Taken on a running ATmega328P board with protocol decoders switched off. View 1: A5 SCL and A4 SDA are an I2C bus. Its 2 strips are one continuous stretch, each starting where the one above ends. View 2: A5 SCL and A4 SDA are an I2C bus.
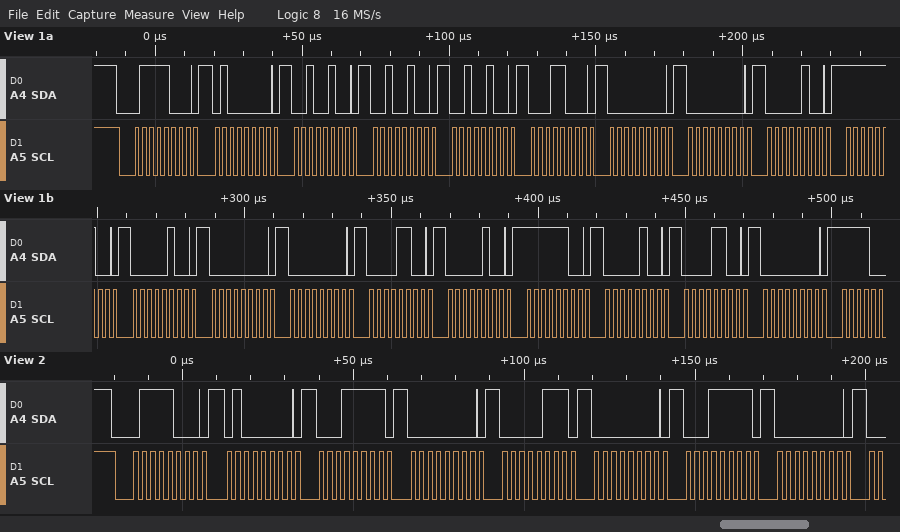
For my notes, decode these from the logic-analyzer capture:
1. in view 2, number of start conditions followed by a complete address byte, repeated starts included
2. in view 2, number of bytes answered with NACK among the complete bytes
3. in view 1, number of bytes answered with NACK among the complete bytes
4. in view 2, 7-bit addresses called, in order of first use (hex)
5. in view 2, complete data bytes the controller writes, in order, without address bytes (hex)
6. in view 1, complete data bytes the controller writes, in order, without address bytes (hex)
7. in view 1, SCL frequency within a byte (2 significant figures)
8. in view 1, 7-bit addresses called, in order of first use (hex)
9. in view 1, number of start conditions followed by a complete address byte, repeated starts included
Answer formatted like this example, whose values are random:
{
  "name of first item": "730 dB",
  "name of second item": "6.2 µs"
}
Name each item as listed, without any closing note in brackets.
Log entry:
{
  "in view 2, number of start conditions followed by a complete address byte, repeated starts included": "1",
  "in view 2, number of bytes answered with NACK among the complete bytes": "0",
  "in view 1, number of bytes answered with NACK among the complete bytes": "0",
  "in view 2, 7-bit addresses called, in order of first use": "0x3C",
  "in view 2, complete data bytes the controller writes, in order, without address bytes": "40 1F 00 07 00 1F 00",
  "in view 1, complete data bytes the controller writes, in order, without address bytes": "40 24 24 24 18 00 00 04 FC 04 00 00 0C 04 FC 04 0C 00",
  "in view 1, SCL frequency within a byte": "400 kHz",
  "in view 1, 7-bit addresses called, in order of first use": "0x3C",
  "in view 1, number of start conditions followed by a complete address byte, repeated starts included": "1"
}
